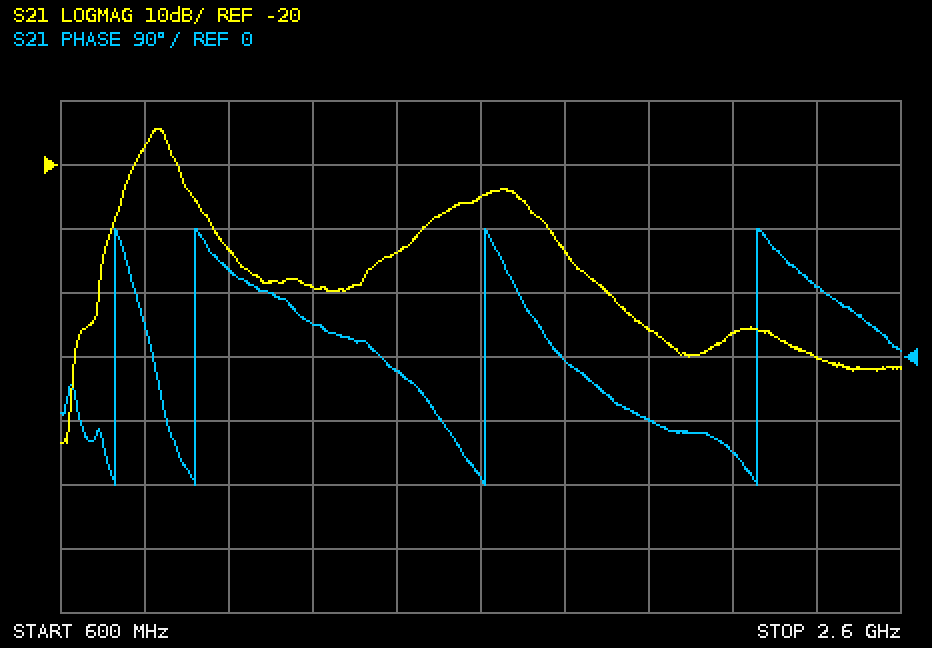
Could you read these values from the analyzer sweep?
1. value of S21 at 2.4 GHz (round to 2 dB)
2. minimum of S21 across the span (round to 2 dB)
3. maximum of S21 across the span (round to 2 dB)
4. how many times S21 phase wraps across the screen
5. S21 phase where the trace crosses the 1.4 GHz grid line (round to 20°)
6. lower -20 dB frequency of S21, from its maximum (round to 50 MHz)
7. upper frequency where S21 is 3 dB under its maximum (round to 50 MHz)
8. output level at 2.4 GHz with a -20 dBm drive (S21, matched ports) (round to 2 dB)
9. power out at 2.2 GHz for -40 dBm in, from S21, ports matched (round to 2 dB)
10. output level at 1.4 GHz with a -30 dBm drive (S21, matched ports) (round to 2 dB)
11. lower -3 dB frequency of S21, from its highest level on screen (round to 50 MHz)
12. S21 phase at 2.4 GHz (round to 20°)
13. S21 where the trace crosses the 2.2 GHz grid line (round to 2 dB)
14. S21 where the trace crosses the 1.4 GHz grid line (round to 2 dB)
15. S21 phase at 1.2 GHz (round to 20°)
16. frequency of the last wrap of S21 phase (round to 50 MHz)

-50 dB
-64 dB
-14 dB
4
-20°
700 MHz
850 MHz
-70 dBm
-86 dBm
-64 dBm
800 MHz
100°
-46 dB
-34 dB
40°
2.25 GHz
